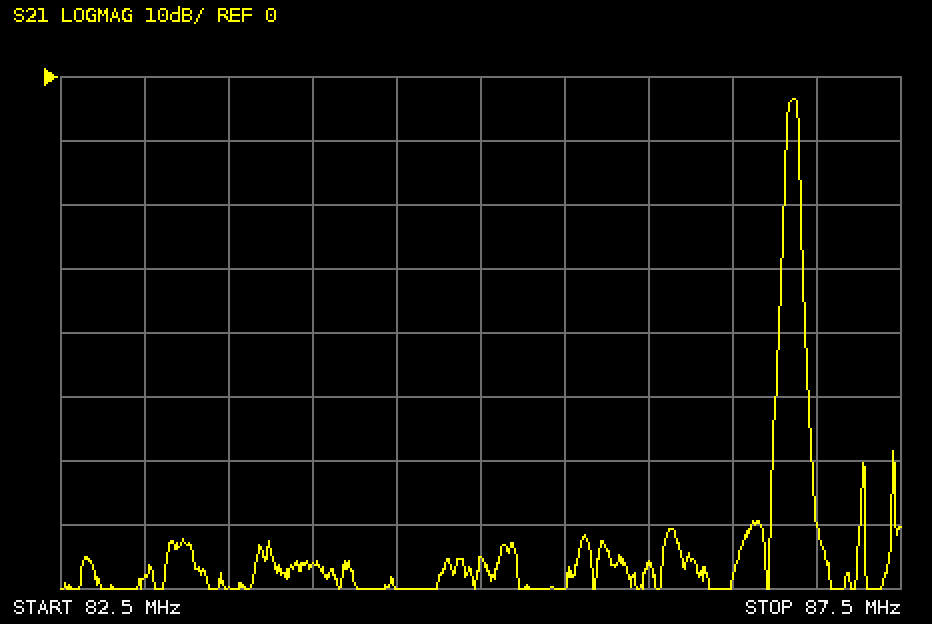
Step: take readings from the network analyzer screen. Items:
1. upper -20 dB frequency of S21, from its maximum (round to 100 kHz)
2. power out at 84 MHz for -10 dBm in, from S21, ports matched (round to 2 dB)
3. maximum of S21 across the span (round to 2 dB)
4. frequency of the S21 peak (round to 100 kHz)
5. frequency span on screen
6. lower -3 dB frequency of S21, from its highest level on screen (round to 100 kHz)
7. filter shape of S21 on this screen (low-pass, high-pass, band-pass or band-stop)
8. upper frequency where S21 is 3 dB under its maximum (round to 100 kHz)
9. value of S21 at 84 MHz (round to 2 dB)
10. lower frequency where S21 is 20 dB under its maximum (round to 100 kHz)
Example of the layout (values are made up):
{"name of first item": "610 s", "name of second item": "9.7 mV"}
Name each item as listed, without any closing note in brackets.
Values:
{"upper -20 dB frequency of S21, from its maximum": "86.9 MHz", "power out at 84 MHz for -10 dBm in, from S21, ports matched": "-86 dBm", "maximum of S21 across the span": "-4 dB", "frequency of the S21 peak": "86.9 MHz", "frequency span on screen": "5 MHz", "lower -3 dB frequency of S21, from its highest level on screen": "86.8 MHz", "filter shape of S21 on this screen": "band-pass", "upper frequency where S21 is 3 dB under its maximum": "86.9 MHz", "value of S21 at 84 MHz": "-76 dB", "lower frequency where S21 is 20 dB under its maximum": "86.8 MHz"}
